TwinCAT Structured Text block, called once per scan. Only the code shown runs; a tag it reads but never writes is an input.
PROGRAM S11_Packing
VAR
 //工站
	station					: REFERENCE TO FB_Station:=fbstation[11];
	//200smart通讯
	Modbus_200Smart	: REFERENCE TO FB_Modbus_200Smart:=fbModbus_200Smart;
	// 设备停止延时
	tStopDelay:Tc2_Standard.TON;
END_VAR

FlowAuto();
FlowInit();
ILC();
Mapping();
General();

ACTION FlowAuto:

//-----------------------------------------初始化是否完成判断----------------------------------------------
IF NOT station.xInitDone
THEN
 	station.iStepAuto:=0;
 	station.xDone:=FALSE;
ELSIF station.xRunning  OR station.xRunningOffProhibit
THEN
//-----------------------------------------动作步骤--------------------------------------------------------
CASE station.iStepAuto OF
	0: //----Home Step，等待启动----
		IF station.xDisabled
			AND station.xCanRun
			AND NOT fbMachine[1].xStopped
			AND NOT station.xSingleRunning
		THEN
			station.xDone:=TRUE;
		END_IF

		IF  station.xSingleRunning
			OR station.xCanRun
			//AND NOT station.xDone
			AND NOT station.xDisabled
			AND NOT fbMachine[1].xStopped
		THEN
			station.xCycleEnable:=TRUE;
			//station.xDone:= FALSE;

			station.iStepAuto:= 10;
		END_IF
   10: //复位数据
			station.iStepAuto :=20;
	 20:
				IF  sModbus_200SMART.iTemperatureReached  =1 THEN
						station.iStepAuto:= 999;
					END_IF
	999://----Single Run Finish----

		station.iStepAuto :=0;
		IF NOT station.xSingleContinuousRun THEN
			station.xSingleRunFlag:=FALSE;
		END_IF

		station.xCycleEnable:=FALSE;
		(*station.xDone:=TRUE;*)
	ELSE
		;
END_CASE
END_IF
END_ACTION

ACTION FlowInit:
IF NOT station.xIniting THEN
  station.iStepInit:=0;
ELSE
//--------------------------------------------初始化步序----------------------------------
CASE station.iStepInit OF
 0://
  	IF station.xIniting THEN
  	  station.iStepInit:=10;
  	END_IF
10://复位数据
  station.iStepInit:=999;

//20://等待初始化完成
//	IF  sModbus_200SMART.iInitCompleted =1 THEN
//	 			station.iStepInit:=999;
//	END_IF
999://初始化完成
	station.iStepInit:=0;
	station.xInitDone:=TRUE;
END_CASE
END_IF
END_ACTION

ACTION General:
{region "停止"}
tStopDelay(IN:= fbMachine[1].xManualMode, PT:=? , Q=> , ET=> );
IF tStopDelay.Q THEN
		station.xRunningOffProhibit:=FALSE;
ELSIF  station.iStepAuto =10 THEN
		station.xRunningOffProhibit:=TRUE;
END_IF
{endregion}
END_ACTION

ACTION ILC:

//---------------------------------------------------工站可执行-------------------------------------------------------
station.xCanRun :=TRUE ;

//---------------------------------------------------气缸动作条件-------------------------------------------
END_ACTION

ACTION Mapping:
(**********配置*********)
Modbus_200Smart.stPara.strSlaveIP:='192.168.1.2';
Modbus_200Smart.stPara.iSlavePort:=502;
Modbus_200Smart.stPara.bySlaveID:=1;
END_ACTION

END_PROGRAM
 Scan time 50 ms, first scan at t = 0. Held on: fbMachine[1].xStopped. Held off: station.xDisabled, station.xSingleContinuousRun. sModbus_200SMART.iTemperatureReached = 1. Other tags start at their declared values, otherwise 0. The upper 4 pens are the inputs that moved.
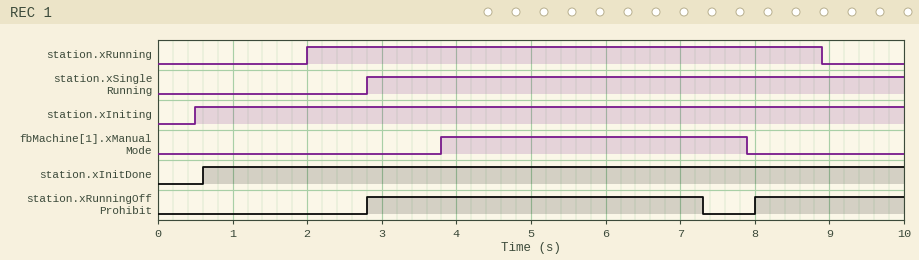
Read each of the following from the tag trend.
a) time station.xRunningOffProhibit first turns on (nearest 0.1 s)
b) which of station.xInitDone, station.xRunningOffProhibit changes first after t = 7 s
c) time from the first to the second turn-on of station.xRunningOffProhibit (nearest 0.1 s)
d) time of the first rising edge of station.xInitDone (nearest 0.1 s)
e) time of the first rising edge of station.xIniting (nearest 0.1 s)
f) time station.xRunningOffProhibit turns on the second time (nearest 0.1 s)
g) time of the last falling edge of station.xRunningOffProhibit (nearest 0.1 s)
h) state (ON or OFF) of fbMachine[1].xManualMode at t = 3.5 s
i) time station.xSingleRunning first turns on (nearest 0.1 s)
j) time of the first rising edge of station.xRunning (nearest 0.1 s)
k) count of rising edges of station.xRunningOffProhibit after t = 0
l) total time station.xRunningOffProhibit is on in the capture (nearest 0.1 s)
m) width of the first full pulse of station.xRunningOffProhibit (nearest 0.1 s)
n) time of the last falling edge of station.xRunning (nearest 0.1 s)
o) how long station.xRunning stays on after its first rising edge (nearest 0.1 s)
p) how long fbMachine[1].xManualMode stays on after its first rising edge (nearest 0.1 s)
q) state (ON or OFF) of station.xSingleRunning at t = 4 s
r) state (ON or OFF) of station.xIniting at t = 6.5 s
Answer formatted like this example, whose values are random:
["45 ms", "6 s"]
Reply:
["2.8 s", "station.xRunningOffProhibit", "5.2 s", "0.6 s", "0.5 s", "8.0 s", "7.3 s", "OFF", "2.8 s", "2.0 s", "2", "6.5 s", "4.5 s", "8.9 s", "6.9 s", "4.1 s", "ON", "ON"]
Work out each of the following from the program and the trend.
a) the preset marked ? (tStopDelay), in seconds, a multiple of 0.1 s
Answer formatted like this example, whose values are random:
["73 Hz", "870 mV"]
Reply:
["3.5 s"]
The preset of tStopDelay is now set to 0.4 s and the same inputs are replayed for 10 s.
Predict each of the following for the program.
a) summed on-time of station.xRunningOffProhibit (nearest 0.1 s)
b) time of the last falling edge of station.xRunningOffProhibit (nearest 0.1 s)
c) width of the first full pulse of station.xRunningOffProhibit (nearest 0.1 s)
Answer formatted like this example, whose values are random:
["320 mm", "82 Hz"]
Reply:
["3.4 s", "4.2 s", "1.4 s"]
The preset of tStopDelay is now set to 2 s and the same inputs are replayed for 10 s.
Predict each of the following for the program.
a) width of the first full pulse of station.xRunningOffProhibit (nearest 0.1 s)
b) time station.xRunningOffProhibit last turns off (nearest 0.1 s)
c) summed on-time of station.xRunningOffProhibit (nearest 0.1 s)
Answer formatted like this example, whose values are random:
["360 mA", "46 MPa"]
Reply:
["3.0 s", "5.8 s", "5.0 s"]
